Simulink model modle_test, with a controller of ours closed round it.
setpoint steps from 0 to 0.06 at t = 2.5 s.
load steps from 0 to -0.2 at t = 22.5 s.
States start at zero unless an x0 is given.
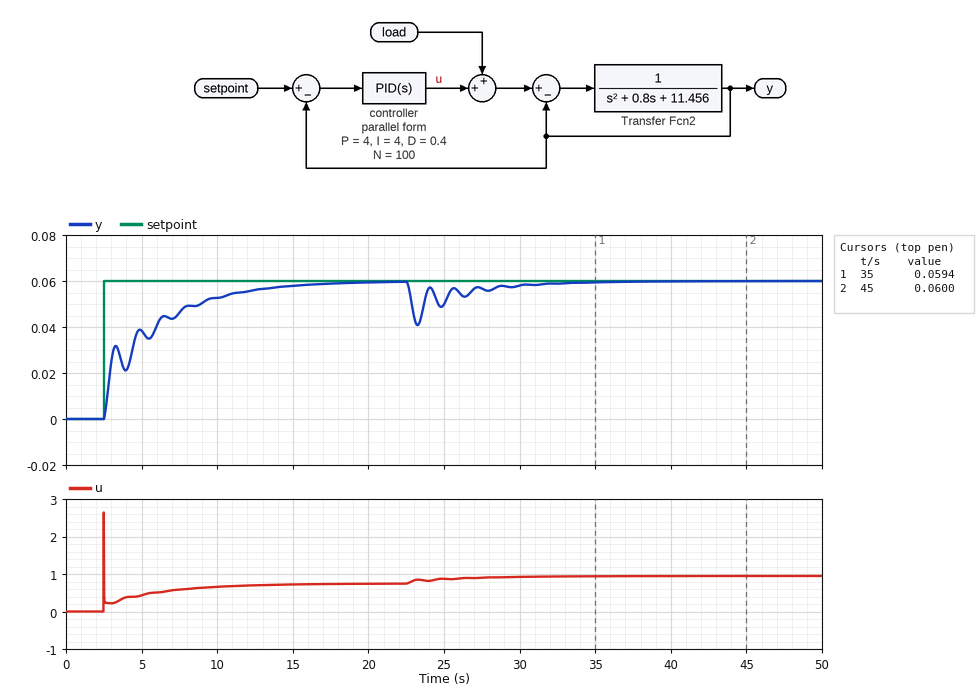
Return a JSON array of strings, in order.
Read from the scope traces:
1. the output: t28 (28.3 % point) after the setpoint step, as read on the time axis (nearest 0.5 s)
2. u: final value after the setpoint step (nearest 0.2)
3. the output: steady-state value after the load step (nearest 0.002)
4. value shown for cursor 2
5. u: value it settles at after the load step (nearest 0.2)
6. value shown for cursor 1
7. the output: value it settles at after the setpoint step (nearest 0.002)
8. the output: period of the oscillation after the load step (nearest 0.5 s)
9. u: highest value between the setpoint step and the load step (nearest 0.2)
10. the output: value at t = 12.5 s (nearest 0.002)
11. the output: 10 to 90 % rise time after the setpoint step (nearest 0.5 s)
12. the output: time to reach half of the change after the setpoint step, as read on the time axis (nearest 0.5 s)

["3.0 s", "0.8", "0.060", "0.0600", "1.0", "0.0594", "0.060", "1.5 s", "2.6", "0.056", "8.0 s", "3.0 s"]
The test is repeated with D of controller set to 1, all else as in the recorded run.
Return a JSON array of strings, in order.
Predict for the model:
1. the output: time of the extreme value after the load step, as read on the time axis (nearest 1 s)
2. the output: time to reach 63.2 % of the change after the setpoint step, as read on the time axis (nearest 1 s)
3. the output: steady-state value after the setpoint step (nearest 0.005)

["23 s", "6 s", "0.060"]
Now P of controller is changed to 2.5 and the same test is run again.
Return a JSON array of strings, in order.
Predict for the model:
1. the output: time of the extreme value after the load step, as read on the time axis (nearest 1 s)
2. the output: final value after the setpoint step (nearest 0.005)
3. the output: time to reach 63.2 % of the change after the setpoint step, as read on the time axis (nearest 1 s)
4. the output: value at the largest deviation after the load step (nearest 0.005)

["23 s", "0.060", "6 s", "0.040"]
